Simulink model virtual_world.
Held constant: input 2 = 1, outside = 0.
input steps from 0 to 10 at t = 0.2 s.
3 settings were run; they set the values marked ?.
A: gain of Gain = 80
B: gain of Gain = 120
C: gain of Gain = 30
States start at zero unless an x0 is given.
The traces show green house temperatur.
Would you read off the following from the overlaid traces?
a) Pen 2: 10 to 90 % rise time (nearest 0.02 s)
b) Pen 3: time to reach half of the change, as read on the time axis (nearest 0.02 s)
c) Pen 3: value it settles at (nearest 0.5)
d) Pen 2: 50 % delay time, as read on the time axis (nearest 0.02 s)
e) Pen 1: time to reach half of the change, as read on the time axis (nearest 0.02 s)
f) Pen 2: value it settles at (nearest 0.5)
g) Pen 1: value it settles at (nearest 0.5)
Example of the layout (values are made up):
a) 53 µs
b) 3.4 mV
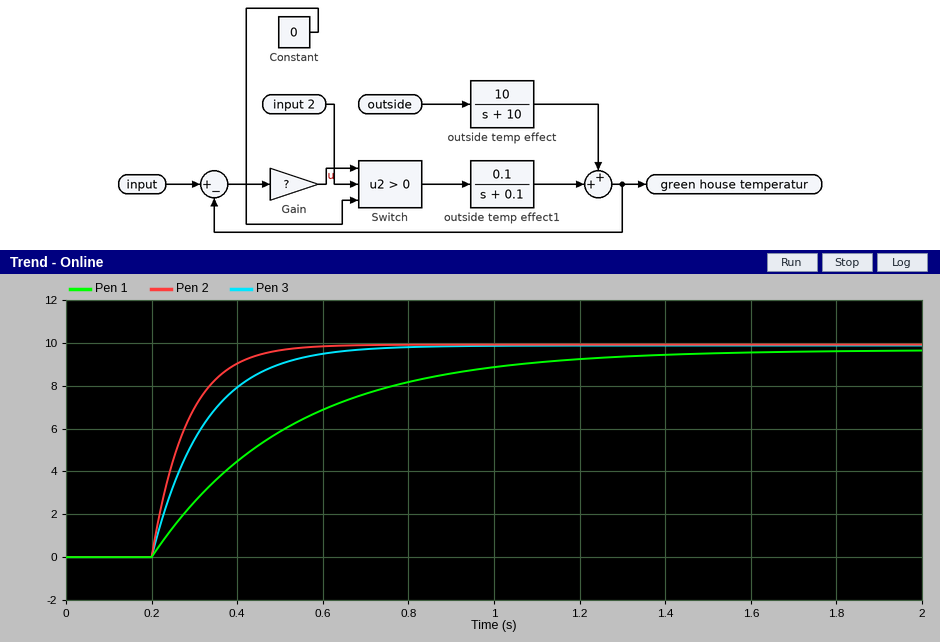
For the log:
a) 0.18 s
b) 0.28 s
c) 10.0
d) 0.26 s
e) 0.42 s
f) 10.0
g) 9.5
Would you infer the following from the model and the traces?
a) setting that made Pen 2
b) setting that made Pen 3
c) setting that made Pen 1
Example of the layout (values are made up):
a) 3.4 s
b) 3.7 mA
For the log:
a) B
b) A
c) C
